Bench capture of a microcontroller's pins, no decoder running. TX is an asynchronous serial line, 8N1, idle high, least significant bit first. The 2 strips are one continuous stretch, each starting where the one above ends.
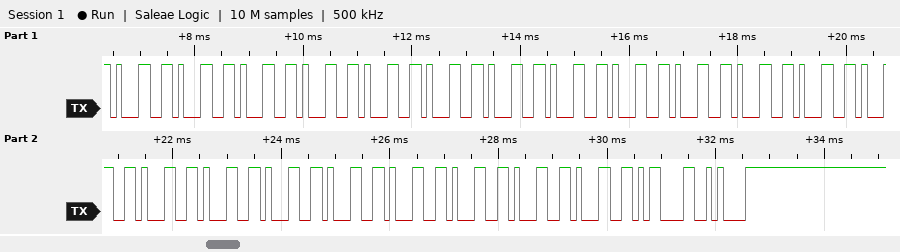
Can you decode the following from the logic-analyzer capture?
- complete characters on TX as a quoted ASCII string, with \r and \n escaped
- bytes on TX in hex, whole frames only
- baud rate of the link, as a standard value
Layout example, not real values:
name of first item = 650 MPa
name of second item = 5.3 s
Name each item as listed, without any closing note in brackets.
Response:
complete characters on TX as a quoted ASCII string, with \r and \n escaped = "111111111111111111111\r\n"
bytes on TX in hex, whole frames only = 31 31 31 31 31 31 31 31 31 31 31 31 31 31 31 31 31 31 31 31 31 0D 0A
baud rate of the link, as a standard value = 9600 baud
